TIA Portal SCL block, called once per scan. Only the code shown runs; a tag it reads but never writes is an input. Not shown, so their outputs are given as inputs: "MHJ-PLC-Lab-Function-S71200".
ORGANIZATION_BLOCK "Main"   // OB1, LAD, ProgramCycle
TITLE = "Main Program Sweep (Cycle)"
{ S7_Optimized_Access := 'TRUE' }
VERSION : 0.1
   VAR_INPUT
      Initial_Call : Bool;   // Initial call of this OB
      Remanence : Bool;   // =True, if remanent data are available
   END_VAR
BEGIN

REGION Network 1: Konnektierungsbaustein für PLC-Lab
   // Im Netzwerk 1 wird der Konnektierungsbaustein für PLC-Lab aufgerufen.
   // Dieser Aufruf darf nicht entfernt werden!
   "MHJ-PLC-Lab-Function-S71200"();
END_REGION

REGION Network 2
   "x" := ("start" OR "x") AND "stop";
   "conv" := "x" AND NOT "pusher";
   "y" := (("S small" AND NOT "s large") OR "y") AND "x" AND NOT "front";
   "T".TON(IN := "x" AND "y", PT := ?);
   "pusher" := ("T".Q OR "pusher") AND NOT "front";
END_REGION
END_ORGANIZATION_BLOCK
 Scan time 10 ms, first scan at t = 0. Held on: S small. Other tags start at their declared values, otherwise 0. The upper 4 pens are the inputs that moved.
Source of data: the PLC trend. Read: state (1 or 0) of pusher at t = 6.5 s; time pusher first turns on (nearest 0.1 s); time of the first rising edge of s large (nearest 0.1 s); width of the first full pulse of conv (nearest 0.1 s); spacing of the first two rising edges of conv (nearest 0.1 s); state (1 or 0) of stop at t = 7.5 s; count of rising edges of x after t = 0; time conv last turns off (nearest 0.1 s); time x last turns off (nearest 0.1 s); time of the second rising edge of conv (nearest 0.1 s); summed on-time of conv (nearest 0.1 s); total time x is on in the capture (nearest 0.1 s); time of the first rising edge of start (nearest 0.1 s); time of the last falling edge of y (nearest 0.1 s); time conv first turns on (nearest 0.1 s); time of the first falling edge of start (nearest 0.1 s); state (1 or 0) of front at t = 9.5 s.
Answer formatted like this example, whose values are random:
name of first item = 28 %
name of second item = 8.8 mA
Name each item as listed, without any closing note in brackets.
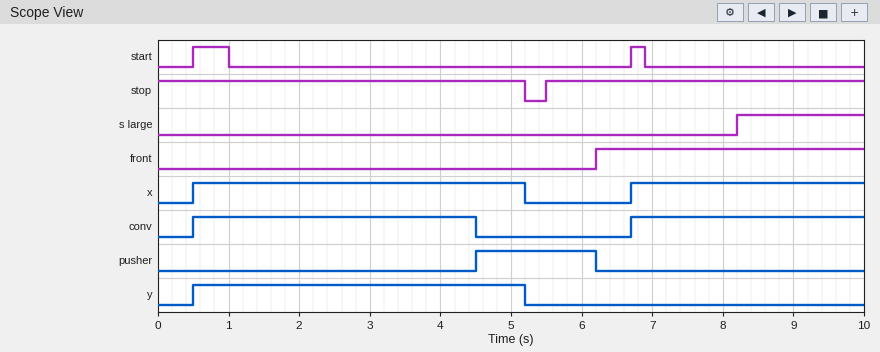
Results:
state (1 or 0) of pusher at t = 6.5 s = 0
time pusher first turns on = 4.5 s
time of the first rising edge of s large = 8.2 s
width of the first full pulse of conv = 4.0 s
spacing of the first two rising edges of conv = 6.2 s
state (1 or 0) of stop at t = 7.5 s = 1
count of rising edges of x after t = 0 = 2
time conv last turns off = 4.5 s
time x last turns off = 5.2 s
time of the second rising edge of conv = 6.7 s
summed on-time of conv = 7.3 s
total time x is on in the capture = 8.0 s
time of the first rising edge of start = 0.5 s
time of the last falling edge of y = 5.2 s
time conv first turns on = 0.5 s
time of the first falling edge of start = 1.0 s
state (1 or 0) of front at t = 9.5 s = 1
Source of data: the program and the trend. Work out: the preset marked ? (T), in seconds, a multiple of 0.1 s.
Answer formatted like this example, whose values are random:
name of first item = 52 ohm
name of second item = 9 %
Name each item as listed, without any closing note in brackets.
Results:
the preset marked ? (T), in seconds, a multiple of 0.1 s = 4.0 s
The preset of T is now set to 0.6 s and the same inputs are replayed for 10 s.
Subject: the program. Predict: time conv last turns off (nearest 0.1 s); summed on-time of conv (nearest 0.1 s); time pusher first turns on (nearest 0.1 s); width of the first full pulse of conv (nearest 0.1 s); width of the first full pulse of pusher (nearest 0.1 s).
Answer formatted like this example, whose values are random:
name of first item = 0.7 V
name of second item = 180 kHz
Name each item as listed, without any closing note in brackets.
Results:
time conv last turns off = 1.1 s
summed on-time of conv = 3.9 s
time pusher first turns on = 1.1 s
width of the first full pulse of conv = 0.6 s
width of the first full pulse of pusher = 5.1 s
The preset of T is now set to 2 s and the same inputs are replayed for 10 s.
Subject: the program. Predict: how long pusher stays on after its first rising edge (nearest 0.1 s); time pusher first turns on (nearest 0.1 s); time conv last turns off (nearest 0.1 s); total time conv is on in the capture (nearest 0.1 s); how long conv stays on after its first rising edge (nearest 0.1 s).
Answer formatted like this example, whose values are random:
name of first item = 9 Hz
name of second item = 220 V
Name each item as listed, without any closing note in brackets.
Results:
how long pusher stays on after its first rising edge = 3.7 s
time pusher first turns on = 2.5 s
time conv last turns off = 2.5 s
total time conv is on in the capture = 5.3 s
how long conv stays on after its first rising edge = 2.0 s
